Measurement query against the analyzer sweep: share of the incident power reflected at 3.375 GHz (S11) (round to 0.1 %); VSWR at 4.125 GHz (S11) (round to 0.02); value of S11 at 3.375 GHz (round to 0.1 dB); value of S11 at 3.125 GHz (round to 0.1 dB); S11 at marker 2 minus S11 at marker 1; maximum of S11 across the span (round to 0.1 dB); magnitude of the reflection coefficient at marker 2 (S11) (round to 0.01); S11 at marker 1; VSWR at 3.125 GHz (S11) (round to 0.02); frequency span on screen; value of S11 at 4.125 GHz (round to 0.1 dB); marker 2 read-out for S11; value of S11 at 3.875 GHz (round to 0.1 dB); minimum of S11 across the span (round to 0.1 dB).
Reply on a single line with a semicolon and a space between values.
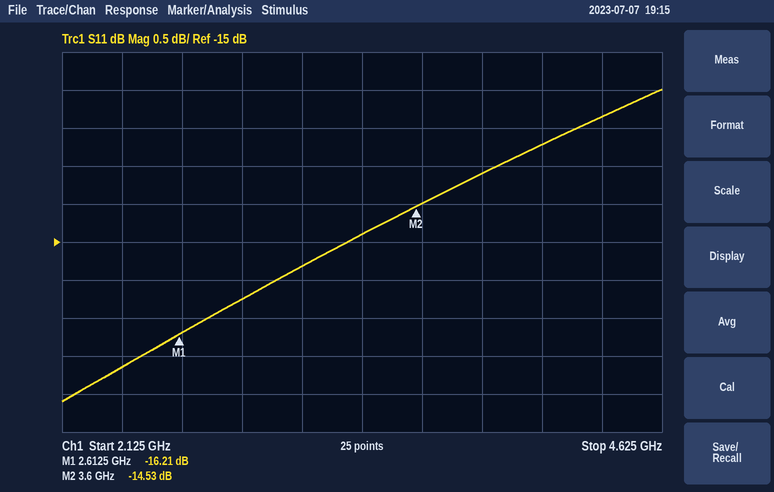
3.2 %; 1.52; -14.9 dB; -15.3 dB; 1.68 dB; -13.0 dB; 0.19; -16.21 dB; 1.42; 2.5 GHz; -13.7 dB; -14.53 dB; -14.1 dB; -17.1 dB
